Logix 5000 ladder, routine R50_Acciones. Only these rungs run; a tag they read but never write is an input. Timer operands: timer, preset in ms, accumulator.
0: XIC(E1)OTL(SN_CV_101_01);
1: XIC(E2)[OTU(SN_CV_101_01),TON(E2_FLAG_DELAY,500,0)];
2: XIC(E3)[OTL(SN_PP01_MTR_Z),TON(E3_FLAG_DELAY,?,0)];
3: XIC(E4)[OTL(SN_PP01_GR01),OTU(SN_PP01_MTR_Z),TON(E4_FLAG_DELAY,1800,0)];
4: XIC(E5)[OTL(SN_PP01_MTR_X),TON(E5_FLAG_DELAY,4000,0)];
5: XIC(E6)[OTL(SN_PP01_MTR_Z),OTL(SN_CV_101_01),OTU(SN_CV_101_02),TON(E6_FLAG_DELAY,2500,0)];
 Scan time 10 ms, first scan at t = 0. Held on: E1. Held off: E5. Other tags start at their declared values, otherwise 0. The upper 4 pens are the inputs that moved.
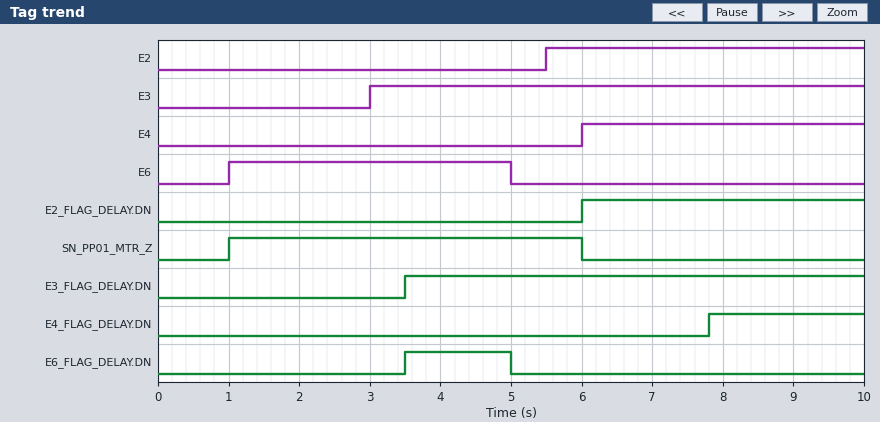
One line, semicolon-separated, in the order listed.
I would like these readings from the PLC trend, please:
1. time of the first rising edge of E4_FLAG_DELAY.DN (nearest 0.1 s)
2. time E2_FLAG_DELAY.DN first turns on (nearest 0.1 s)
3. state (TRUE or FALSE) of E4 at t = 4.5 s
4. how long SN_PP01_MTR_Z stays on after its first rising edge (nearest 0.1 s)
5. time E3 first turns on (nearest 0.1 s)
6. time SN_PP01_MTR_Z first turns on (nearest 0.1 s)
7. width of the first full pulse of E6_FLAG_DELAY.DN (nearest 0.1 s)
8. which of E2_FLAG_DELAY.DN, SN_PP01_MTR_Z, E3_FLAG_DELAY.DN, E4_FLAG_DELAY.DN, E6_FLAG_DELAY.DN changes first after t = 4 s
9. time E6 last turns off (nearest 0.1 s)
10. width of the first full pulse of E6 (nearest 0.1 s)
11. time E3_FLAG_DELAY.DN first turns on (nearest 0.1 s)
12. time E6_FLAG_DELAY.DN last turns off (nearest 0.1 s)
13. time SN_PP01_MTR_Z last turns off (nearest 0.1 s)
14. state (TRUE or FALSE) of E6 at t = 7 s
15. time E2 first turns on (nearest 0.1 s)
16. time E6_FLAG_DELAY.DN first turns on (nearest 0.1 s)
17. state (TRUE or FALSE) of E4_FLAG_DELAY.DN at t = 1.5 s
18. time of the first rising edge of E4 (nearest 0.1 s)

7.8 s; 6.0 s; FALSE; 5.0 s; 3.0 s; 1.0 s; 1.5 s; E6_FLAG_DELAY.DN; 5.0 s; 4.0 s; 3.5 s; 5.0 s; 6.0 s; FALSE; 5.5 s; 3.5 s; FALSE; 6.0 s
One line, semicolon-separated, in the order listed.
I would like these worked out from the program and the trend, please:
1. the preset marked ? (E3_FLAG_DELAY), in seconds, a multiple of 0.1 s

0.5 s
